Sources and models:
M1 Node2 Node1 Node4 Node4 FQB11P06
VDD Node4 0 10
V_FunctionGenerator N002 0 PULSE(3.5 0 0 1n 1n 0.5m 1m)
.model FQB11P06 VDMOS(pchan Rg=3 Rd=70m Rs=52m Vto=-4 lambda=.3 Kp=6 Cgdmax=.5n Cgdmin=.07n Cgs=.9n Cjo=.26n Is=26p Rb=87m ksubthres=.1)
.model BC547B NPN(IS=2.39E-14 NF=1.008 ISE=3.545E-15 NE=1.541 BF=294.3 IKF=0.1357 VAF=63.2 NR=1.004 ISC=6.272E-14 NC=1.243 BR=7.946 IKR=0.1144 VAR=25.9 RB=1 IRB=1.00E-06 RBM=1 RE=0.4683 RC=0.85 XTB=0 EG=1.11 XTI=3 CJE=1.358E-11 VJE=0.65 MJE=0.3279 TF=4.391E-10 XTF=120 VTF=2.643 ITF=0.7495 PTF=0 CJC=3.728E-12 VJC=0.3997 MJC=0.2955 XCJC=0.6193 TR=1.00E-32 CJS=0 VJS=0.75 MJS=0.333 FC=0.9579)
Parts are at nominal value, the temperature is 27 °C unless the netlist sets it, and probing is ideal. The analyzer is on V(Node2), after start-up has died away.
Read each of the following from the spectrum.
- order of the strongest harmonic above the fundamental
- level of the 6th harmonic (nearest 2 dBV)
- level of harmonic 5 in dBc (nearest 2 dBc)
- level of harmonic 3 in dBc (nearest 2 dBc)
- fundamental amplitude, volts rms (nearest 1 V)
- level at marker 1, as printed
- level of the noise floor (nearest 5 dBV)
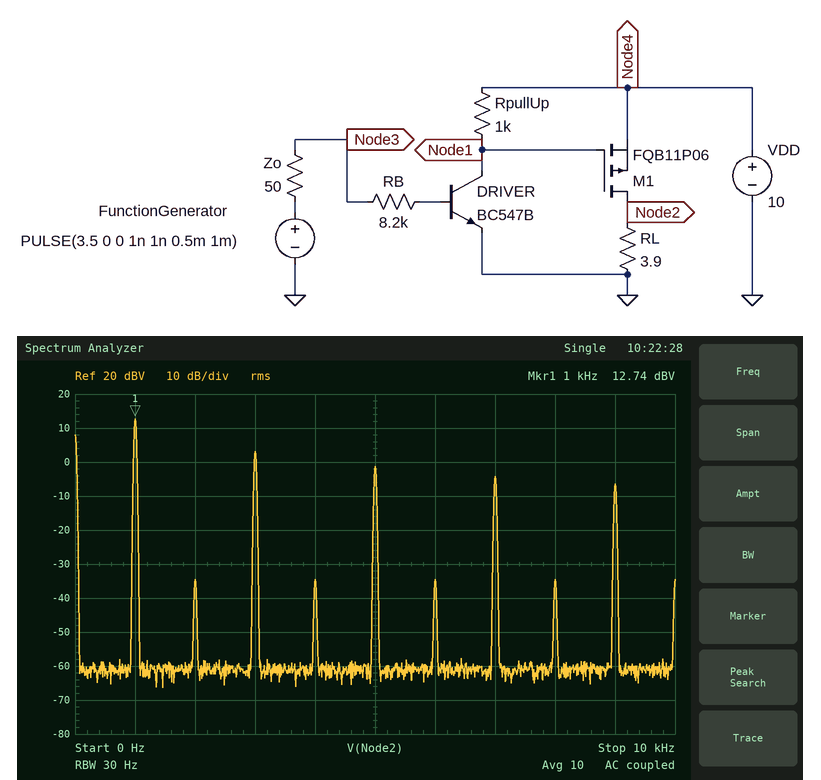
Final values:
3
-34 dBV
-14 dBc
-10 dBc
4 V
12.74 dBV
-60 dBV
